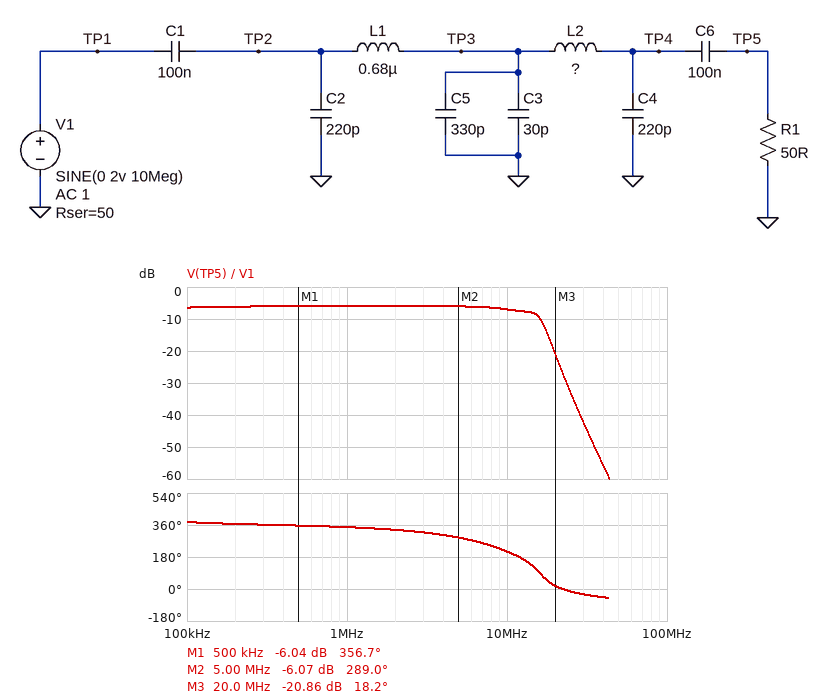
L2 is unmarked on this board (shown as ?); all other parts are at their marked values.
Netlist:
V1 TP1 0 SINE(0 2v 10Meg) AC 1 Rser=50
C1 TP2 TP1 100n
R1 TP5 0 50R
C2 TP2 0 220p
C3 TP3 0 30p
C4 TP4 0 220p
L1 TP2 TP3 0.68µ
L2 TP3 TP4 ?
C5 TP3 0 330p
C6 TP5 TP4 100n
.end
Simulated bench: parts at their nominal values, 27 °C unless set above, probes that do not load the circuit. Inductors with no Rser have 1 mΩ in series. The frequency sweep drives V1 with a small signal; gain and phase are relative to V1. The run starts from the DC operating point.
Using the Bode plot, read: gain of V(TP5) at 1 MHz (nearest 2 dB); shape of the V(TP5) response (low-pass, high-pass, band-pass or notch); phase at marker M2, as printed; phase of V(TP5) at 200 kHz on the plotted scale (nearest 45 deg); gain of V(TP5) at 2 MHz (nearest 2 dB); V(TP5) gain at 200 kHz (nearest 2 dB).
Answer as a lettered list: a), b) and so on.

a) -6 dB
b) low-pass
c) 289.0 deg
d) 360 deg
e) -6 dB
f) -6 dB
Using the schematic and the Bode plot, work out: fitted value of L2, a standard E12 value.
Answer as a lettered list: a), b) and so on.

a) 1.2 µH
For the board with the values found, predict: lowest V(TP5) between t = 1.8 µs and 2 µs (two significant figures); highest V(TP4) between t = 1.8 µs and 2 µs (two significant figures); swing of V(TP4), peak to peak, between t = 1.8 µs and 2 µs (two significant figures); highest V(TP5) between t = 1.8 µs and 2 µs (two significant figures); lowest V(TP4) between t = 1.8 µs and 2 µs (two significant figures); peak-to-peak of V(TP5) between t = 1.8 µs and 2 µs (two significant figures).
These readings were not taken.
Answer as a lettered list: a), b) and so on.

a) -900 mV
b) 890 mV
c) 1.8 V
d) 890 mV
e) -890 mV
f) 1.8 V
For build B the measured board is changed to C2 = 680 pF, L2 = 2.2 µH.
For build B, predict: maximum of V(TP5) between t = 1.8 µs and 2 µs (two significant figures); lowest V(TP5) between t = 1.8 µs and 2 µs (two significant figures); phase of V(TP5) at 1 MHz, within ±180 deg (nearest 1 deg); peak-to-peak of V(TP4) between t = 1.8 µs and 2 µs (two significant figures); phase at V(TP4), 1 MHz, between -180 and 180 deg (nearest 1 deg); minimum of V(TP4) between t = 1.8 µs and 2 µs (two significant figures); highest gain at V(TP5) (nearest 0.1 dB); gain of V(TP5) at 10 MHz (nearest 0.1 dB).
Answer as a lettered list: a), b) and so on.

a) 410 mV
b) -420 mV
c) -20 deg
d) 830 mV
e) -22 deg
f) -410 mV
g) -6.0 dB
h) -13.7 dB
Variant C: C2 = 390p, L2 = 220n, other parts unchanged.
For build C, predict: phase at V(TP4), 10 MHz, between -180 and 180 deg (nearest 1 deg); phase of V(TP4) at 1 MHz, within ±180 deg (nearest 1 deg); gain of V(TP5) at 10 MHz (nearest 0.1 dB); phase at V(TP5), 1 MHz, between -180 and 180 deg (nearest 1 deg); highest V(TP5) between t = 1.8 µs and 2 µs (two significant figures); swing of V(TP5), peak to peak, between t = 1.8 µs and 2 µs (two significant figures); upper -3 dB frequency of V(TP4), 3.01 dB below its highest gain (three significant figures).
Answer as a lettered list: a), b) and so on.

a) -118 deg
b) -12 deg
c) -6.1 dB
d) -10 deg
e) 990 mV
f) 2.0 V
g) 14.1 MHz
